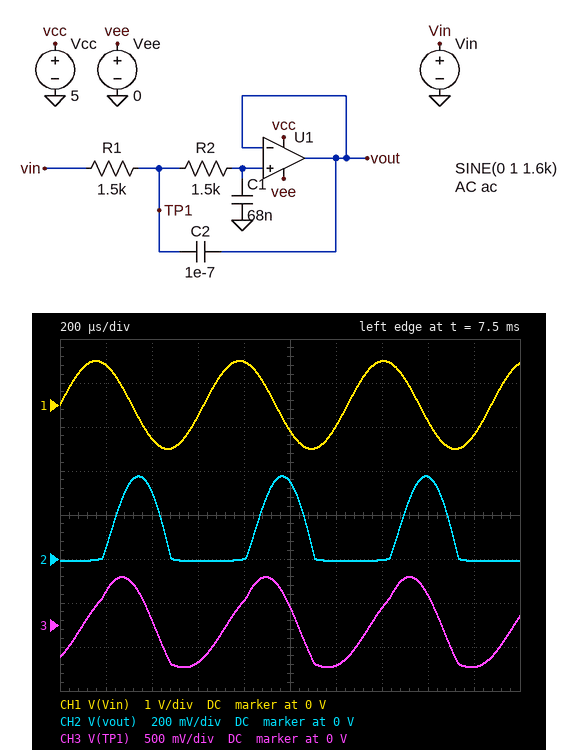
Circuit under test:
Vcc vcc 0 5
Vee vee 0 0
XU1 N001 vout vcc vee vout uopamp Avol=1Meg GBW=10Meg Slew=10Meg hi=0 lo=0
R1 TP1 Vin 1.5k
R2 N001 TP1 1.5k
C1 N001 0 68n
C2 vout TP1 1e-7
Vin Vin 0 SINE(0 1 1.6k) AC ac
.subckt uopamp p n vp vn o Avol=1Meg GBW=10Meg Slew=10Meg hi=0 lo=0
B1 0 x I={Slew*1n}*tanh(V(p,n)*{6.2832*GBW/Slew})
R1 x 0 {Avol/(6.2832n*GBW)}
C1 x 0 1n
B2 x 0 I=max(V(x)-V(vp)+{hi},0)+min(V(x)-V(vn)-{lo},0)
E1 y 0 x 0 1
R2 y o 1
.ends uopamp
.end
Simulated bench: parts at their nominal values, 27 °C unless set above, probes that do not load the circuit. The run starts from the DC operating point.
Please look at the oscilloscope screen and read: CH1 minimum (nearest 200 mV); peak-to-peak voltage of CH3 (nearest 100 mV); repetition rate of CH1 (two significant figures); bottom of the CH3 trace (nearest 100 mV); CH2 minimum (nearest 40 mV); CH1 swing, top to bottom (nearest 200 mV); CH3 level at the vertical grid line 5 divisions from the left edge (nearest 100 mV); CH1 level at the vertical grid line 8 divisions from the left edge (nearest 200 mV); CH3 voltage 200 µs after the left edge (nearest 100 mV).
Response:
-1.0 V
1.0 V
1.6 kHz
-500 mV
0 V
2.0 V
200 mV
-400 mV
400 mV
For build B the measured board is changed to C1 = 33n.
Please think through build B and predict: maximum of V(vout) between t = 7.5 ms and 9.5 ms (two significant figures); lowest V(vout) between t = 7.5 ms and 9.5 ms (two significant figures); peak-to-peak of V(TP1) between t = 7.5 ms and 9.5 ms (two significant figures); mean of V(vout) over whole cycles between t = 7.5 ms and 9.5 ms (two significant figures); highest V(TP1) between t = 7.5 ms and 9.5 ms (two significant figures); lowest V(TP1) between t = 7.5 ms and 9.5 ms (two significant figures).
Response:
670 mV
-10 mV
1.3 V
180 mV
770 mV
-570 mV
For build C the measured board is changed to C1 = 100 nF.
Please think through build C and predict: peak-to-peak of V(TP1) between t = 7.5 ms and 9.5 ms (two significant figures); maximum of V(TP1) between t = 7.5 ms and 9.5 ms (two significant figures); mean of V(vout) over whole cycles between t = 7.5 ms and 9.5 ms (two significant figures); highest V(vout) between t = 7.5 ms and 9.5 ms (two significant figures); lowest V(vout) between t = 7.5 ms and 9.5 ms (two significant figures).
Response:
930 mV
470 mV
77 mV
260 mV
-8.7 mV
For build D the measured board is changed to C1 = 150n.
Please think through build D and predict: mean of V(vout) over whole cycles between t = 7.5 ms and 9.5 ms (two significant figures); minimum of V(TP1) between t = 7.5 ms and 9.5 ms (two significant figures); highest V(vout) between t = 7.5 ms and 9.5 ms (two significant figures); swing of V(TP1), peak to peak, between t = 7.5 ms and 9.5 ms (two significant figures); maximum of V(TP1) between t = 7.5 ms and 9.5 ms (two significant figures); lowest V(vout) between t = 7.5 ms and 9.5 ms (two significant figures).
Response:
53 mV
-440 mV
180 mV
870 mV
430 mV
-7.3 mV
